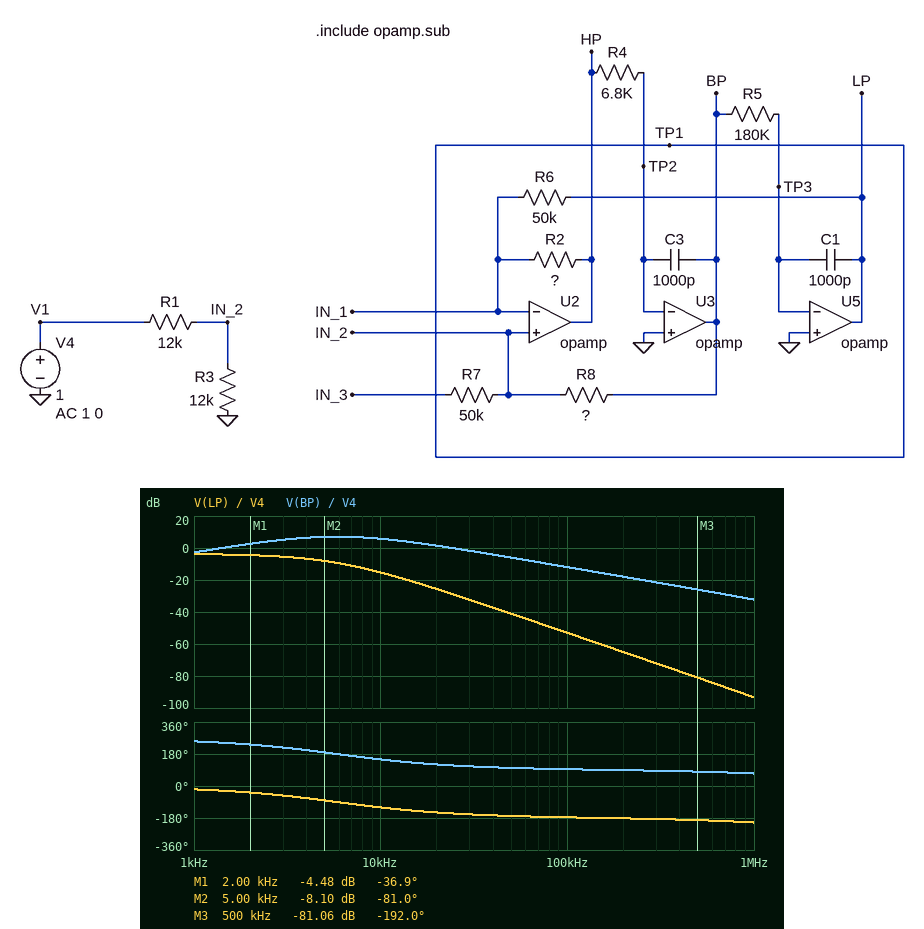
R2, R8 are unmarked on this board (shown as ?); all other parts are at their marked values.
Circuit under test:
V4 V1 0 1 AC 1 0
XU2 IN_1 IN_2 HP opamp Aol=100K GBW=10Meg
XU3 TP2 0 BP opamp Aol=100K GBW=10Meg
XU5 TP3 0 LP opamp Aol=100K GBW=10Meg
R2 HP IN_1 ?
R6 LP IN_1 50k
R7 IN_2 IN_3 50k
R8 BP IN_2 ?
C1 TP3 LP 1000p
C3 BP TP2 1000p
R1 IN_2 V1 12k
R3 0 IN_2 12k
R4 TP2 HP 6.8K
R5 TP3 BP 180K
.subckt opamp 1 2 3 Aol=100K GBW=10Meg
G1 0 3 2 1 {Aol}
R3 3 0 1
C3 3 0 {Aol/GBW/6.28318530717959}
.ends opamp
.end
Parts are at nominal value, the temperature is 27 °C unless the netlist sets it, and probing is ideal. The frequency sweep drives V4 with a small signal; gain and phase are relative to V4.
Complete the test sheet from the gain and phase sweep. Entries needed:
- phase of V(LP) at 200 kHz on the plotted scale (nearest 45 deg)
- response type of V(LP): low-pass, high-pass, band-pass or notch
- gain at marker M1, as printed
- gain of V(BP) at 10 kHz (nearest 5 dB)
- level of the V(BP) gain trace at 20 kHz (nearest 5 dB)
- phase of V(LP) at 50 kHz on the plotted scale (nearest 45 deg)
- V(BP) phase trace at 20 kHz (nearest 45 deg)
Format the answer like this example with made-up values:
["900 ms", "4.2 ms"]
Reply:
["-180 deg", "low-pass", "-4.48 dB", "5 dB", "0 dB", "-180 deg", "135 deg"]
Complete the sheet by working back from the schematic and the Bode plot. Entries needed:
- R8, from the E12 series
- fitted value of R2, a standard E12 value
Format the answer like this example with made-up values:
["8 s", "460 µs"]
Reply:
["27 kΩ", "82 kΩ"]
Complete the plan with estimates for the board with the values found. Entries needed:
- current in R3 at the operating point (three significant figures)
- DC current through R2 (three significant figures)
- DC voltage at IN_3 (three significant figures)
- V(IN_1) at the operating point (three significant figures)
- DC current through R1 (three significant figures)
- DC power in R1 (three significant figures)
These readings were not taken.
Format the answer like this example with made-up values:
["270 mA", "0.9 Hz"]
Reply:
["34.1 µA", "4.99 µA", "409 mV", "409 mV", "49.2 µA", "29.1 µW"]
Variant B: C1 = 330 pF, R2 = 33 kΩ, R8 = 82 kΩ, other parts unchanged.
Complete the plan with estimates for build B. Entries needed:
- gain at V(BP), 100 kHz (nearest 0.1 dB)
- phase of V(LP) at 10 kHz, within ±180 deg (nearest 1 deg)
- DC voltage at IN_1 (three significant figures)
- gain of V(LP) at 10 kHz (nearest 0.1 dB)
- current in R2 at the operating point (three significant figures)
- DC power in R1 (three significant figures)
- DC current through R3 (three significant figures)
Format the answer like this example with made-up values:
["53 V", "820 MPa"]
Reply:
["-14.8 dB", "-156 deg", "466 mV", "-2.5 dB", "14.1 µA", "23.8 µW", "38.8 µA"]
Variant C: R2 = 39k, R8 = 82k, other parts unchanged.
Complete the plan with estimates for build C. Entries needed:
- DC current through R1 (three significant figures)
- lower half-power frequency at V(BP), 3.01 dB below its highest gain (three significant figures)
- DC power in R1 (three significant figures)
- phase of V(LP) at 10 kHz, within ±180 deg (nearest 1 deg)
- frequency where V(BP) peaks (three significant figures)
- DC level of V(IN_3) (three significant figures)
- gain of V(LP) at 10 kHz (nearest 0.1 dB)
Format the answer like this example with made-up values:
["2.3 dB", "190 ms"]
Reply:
["44.5 µA", "2.84 kHz", "23.8 µW", "-162 deg", "4.01 kHz", "466 mV", "-14.3 dB"]
